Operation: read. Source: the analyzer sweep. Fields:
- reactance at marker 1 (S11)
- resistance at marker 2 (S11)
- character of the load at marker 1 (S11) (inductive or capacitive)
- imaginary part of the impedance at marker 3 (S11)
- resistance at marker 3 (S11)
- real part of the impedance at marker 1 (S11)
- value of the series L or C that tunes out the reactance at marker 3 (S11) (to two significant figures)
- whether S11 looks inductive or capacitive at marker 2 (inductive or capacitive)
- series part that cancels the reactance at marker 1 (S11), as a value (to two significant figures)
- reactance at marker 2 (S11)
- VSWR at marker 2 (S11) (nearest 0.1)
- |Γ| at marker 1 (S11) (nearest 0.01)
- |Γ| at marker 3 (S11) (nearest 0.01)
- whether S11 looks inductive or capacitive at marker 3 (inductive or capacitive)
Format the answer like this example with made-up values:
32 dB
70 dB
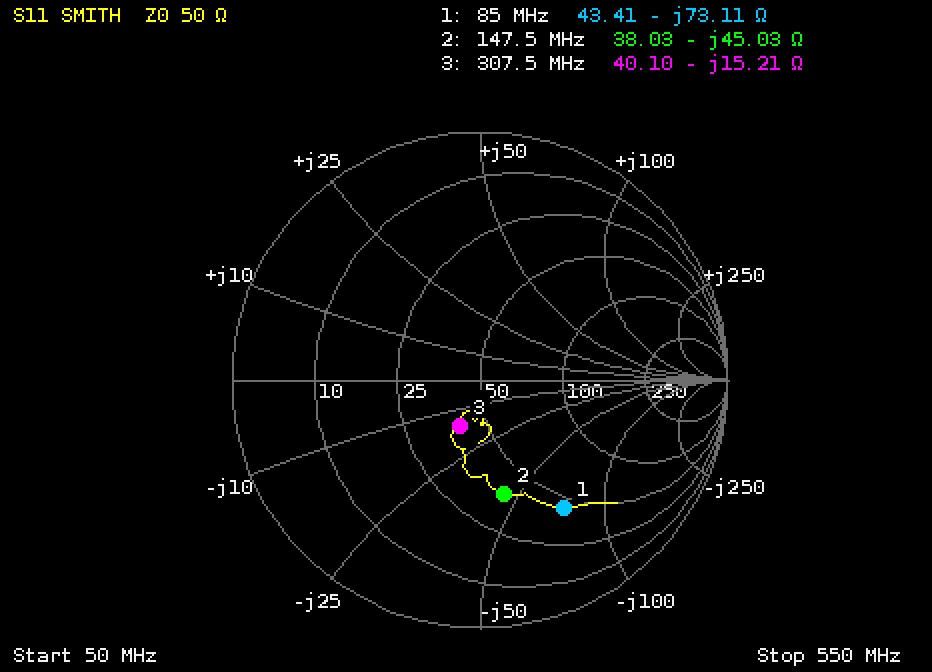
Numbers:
-73.11 Ω
38.03 Ω
capacitive
-15.21 Ω
40.10 Ω
43.41 Ω
7.9 nH
capacitive
140 nH
-45.03 Ω
2.8
0.62
0.20
capacitive
